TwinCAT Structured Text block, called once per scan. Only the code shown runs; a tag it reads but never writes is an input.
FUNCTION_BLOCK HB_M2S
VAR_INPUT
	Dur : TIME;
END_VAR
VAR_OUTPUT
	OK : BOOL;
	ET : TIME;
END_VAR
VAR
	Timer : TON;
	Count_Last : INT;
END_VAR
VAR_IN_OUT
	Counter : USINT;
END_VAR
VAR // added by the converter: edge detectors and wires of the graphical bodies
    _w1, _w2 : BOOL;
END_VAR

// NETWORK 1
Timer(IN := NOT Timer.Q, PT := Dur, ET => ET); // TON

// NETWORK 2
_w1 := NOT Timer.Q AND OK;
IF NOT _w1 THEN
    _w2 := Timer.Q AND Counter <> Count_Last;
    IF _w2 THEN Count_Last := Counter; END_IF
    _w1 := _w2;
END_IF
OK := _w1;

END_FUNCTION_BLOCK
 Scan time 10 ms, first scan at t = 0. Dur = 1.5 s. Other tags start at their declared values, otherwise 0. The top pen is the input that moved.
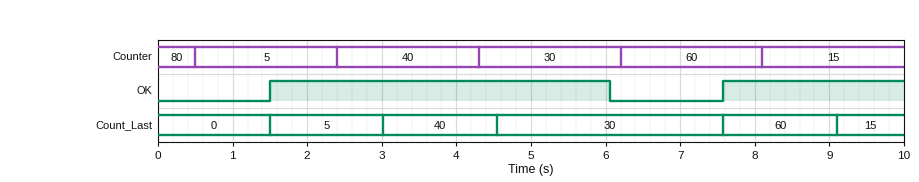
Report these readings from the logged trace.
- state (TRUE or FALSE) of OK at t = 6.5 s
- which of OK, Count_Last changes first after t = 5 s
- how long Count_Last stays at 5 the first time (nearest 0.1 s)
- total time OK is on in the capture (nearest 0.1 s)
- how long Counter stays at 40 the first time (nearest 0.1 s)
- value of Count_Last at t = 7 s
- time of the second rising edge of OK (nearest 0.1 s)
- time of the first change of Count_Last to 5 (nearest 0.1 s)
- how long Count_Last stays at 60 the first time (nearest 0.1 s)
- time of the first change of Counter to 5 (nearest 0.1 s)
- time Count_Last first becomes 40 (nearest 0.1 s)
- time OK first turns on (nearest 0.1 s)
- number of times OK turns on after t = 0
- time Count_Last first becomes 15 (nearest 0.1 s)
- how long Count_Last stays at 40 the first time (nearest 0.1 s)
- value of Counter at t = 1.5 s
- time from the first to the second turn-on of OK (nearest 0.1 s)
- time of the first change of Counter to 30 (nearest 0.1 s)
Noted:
FALSE
OK
1.5 s
7.0 s
1.9 s
30
7.6 s
1.5 s
1.5 s
0.5 s
3.0 s
1.5 s
2
9.1 s
1.5 s
5
6.1 s
4.3 s
